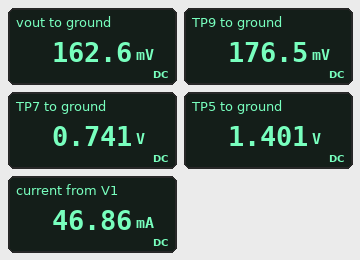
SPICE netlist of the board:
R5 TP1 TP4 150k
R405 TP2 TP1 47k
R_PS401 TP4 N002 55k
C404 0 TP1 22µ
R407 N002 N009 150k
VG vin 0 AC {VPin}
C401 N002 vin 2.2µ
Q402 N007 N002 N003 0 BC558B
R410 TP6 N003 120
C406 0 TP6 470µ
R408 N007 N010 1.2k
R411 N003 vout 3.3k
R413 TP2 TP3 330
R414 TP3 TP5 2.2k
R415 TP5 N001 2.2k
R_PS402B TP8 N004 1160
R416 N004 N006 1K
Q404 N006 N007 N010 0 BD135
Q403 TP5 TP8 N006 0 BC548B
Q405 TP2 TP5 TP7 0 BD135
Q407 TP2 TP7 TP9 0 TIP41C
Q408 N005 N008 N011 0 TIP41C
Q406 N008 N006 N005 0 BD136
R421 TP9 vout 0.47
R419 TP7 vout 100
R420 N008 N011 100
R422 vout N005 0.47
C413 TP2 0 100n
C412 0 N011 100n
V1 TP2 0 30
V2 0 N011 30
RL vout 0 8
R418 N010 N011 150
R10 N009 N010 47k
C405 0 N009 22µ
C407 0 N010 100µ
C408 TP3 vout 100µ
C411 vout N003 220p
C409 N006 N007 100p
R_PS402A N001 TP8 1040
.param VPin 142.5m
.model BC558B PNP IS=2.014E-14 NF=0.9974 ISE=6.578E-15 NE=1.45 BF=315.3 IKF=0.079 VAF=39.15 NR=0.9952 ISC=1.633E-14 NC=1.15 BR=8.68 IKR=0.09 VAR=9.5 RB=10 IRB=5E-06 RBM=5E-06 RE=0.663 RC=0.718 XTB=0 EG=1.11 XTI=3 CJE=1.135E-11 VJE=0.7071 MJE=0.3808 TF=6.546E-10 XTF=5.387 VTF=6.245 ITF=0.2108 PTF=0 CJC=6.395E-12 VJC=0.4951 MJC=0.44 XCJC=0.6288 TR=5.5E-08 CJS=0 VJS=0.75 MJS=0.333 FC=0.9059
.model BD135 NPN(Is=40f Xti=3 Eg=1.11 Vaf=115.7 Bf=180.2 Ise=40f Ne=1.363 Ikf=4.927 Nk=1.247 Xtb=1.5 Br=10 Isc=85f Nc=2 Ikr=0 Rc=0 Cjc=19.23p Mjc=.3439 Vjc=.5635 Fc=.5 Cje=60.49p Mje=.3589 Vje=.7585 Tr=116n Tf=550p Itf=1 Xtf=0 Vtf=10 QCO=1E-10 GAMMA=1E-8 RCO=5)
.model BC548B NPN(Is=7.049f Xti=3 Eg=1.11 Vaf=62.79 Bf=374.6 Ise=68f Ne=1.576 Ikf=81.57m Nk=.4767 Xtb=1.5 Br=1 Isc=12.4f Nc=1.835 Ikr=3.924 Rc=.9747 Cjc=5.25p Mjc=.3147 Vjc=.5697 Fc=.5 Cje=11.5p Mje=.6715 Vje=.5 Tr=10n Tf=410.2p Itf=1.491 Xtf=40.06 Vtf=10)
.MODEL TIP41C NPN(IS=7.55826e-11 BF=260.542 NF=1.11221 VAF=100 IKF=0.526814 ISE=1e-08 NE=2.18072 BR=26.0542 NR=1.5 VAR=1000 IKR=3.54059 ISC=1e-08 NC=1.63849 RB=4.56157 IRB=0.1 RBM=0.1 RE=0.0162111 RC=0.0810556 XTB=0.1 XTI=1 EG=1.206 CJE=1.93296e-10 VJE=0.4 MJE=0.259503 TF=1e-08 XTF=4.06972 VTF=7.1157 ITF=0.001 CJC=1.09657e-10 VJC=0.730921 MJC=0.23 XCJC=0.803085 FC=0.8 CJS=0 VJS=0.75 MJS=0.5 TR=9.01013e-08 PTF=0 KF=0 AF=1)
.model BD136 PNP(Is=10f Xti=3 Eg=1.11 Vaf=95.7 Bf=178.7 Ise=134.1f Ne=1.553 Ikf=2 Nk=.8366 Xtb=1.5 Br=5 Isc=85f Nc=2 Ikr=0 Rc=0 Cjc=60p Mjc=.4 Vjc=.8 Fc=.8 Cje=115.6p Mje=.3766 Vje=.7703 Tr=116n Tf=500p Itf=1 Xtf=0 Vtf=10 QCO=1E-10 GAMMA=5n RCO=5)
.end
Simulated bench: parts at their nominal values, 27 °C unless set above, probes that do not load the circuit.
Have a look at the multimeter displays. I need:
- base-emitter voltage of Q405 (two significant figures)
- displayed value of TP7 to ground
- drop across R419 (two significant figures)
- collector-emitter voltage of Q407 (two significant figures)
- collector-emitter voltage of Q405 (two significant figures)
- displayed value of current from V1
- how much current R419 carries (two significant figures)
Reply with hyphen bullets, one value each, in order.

- 660 mV
- 0.741 V
- 580 mV
- 30 V
- 29 V
- 46.86 mA
- 5.8 mA
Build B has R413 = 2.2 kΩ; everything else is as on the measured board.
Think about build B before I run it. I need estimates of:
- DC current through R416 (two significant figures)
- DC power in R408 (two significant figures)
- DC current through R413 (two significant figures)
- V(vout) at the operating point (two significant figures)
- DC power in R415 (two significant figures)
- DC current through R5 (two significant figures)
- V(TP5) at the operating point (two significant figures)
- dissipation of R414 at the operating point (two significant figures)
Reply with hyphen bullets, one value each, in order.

- 330 µA
- 370 µW
- 6.6 mA
- -360 mV
- 270 µW
- 130 µA
- 770 mV
- 97 mW
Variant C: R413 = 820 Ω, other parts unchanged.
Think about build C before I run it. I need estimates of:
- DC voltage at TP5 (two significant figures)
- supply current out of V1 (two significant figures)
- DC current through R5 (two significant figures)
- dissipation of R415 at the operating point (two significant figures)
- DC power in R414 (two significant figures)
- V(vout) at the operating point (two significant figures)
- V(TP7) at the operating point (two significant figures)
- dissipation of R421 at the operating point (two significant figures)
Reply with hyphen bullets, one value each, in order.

- 1.2 V
- 28 mA
- 130 µA
- 290 µW
- 200 mW
- -32 mV
- 510 mV
- 75 µW
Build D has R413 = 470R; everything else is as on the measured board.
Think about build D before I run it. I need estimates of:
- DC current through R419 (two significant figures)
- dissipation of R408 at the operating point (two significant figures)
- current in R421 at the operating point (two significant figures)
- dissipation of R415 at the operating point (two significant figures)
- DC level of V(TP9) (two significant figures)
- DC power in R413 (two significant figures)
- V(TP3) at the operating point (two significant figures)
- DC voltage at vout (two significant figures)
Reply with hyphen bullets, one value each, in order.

- 5.7 mA
- 380 µW
- 23 mA
- 300 µW
- 110 mV
- 54 mW
- 25 V
- 100 mV
